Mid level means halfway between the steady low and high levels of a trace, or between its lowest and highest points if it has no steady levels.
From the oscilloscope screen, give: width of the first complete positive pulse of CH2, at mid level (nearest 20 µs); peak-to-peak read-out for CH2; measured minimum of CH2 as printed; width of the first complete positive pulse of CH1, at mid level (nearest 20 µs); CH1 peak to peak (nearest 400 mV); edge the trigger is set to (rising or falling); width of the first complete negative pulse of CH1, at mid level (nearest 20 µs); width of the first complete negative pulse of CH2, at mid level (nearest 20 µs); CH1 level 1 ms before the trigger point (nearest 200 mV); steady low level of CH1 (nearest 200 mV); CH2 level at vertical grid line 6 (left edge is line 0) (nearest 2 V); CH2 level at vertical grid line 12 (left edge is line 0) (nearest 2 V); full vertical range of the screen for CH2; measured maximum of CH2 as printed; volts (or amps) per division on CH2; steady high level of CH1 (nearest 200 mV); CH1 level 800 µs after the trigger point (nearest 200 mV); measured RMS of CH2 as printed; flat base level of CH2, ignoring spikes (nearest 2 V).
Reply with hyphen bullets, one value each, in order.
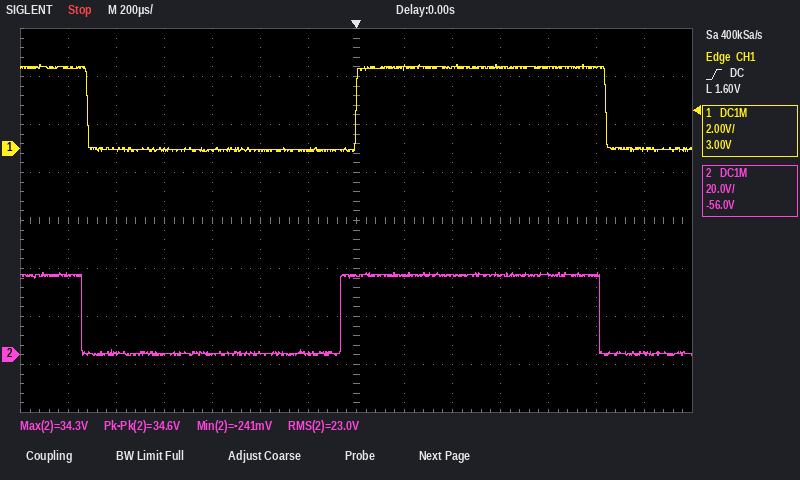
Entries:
- 1.08 ms
- 34.6 V
- -241 mV
- 1.04 ms
- 3.6 V
- rising
- 1.12 ms
- 1.08 ms
- 0.0 V
- 0.0 V
- 0 V
- 34 V
- 160 V
- 34.3 V
- 20 V
- 3.4 V
- 3.4 V
- 23.0 V
- 0 V
